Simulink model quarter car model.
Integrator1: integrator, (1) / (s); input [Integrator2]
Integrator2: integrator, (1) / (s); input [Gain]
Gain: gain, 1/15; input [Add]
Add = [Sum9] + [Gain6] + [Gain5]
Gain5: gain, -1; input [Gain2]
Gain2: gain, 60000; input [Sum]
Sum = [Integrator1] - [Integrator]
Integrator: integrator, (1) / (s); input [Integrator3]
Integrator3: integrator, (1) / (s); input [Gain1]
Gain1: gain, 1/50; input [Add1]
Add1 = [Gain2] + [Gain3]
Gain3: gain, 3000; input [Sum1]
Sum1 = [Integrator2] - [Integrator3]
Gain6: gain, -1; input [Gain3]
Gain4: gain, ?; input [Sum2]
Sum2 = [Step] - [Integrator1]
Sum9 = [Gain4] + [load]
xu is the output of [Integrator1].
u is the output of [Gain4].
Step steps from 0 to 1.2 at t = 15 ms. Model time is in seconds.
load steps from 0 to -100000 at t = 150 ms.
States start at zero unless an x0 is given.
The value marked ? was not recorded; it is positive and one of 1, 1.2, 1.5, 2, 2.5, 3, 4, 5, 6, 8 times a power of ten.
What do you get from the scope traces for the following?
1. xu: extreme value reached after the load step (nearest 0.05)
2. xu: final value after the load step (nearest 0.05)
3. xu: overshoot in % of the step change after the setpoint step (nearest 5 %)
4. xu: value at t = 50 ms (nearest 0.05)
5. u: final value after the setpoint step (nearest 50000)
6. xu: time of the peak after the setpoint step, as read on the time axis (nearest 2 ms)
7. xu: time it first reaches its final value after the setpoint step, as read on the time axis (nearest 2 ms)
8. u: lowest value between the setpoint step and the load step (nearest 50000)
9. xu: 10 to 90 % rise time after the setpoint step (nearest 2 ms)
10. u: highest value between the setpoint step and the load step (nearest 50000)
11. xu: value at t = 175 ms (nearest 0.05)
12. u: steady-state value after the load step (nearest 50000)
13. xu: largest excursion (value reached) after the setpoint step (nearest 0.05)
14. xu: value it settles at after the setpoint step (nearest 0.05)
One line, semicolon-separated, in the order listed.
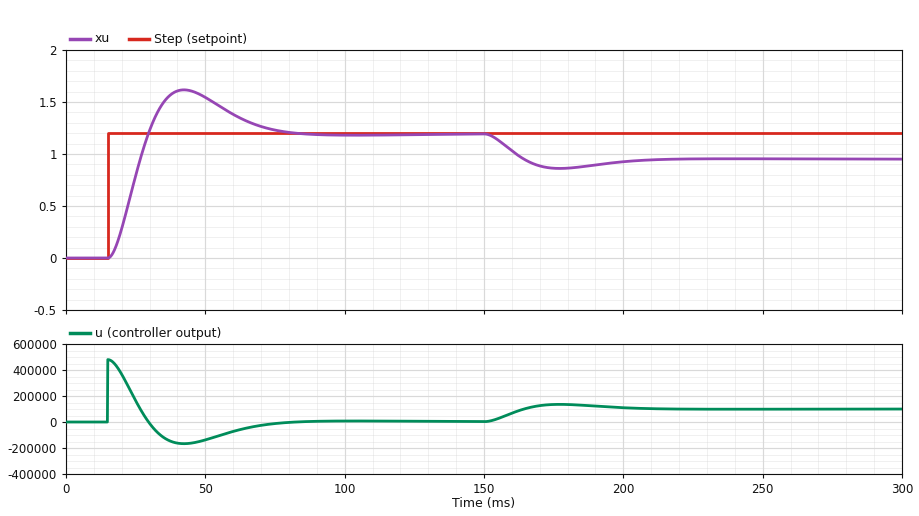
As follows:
0.85; 0.95; 35 %; 1.55; 0; 42 ms; 30 ms; -150000; 10 ms; 500000; 0.85; 100000; 1.60; 1.20
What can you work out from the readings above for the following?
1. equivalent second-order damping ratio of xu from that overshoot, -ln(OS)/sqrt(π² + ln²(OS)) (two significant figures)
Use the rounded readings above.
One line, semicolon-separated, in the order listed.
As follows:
0.32
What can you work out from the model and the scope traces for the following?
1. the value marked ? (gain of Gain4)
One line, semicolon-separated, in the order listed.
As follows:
400000
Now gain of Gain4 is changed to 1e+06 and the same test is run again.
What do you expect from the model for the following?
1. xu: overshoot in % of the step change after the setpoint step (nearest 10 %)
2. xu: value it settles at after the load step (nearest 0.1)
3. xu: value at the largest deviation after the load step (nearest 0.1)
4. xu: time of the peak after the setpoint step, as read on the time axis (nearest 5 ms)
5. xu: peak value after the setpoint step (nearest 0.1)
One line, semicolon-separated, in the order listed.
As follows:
40 %; 1.1; 1.1; 30 ms; 1.7
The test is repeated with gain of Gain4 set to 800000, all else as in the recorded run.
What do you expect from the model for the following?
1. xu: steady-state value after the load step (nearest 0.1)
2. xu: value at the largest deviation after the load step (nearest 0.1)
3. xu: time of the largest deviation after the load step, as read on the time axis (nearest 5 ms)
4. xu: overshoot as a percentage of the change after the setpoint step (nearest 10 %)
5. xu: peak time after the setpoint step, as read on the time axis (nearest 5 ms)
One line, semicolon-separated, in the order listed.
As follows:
1.1; 1.0; 165 ms; 40 %; 30 ms
